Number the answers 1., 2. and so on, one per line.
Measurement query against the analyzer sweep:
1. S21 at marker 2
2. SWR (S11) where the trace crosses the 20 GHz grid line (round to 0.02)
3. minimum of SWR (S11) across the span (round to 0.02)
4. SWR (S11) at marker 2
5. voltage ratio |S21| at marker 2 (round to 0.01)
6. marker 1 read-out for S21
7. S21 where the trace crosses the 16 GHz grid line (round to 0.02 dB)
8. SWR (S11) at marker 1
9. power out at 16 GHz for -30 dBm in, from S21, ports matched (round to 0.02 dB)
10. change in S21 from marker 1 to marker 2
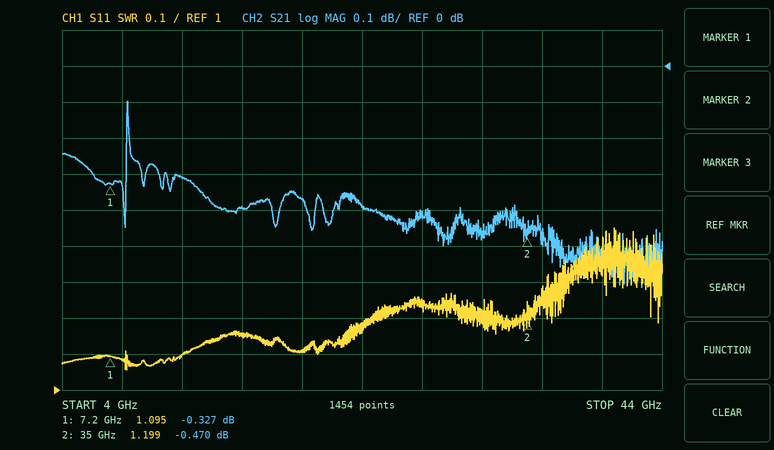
1. -0.470 dB
2. 1.10
3. 1.06
4. 1.199
5. 0.95
6. -0.327 dB
7. -0.40 dB
8. 1.095
9. -30.40 dBm
10. -0.143 dB
